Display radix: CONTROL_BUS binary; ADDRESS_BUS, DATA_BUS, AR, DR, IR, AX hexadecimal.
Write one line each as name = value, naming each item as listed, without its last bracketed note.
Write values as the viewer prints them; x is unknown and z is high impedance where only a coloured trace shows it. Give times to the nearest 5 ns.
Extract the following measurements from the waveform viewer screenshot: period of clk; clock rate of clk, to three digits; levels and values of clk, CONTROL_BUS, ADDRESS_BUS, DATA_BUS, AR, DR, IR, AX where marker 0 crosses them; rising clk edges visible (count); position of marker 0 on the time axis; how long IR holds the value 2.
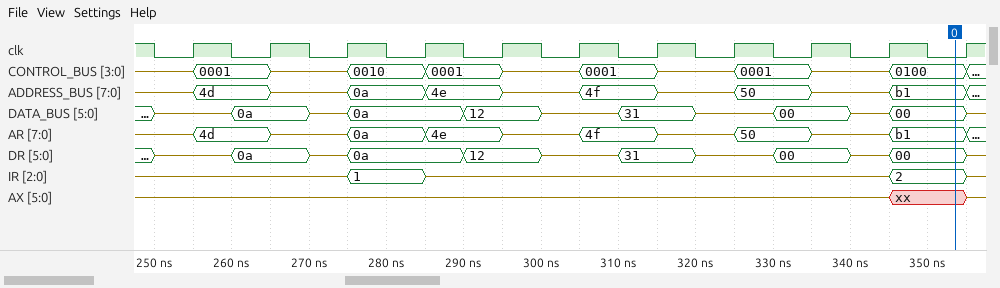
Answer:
period of clk = 10 ns
clock rate of clk, to three digits = 100 MHz
levels and values of clk, CONTROL_BUS, ADDRESS_BUS, DATA_BUS, AR, DR, IR, AX where marker 0 crosses them = clk=0, CONTROL_BUS=0100, ADDRESS_BUS=b1, DATA_BUS=00, AR=b1, DR=00, IR=2, AX=xx
rising clk edges visible = 11
position of marker 0 on the time axis = 355 ns
how long IR holds the value 2 = 10 ns
